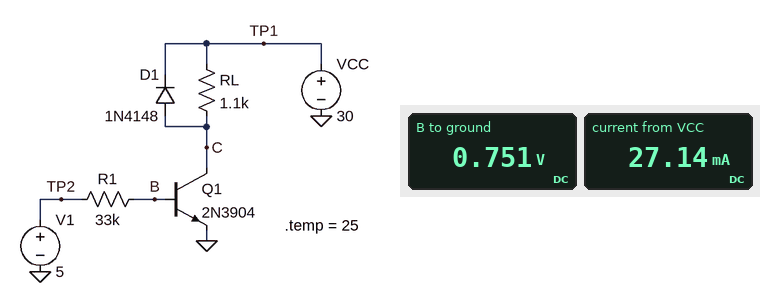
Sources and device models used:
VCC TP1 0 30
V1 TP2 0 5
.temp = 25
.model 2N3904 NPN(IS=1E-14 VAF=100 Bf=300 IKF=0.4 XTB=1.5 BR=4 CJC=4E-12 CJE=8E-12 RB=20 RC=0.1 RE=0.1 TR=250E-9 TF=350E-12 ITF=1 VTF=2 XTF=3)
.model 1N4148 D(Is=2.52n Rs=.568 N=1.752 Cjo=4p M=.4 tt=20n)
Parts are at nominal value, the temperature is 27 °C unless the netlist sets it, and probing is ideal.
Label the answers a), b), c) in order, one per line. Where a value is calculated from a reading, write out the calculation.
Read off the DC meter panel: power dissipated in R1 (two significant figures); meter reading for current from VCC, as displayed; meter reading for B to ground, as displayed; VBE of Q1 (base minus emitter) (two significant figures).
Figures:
a) (5 V - 751 mV)^2 / 33 kΩ = 550 µW
b) 27.14 mA
c) 0.751 V
d) 751 mV = 750 mV
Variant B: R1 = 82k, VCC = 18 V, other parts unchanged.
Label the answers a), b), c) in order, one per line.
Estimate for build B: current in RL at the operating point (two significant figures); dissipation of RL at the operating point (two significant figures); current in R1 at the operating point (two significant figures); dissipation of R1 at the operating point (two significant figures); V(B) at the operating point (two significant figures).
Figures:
a) 15 mA
b) 250 mW
c) 52 µA
d) 220 µW
e) 730 mV
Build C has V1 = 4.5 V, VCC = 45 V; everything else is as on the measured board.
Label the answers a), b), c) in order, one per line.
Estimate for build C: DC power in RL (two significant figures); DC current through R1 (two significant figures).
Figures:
a) 1.2 W
b) 110 µA
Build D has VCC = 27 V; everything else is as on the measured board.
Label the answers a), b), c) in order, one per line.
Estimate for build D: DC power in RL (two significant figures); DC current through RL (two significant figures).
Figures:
a) 660 mW
b) 24 mA
